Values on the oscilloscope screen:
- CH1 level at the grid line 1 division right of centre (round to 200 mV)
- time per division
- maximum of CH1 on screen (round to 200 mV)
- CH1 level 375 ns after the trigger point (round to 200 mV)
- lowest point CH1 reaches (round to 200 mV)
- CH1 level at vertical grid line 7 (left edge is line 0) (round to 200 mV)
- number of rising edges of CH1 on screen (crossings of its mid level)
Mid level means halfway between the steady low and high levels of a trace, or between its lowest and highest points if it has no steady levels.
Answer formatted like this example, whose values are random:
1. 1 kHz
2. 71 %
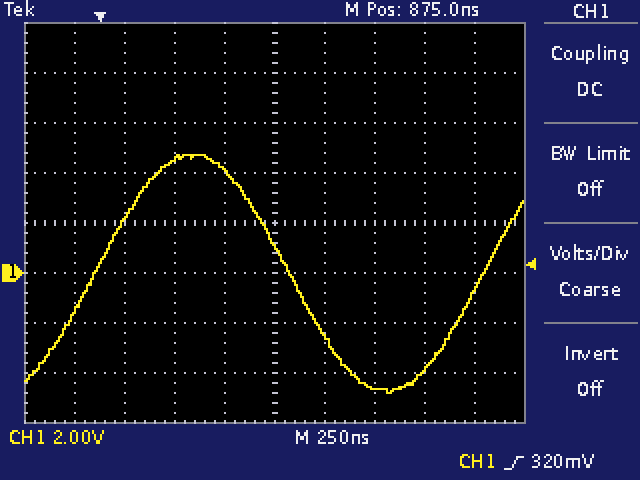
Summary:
1. -2.4 V
2. 250 ns
3. 4.8 V
4. 4.6 V
5. -4.8 V
6. -4.6 V
7. 2
